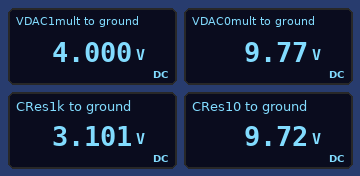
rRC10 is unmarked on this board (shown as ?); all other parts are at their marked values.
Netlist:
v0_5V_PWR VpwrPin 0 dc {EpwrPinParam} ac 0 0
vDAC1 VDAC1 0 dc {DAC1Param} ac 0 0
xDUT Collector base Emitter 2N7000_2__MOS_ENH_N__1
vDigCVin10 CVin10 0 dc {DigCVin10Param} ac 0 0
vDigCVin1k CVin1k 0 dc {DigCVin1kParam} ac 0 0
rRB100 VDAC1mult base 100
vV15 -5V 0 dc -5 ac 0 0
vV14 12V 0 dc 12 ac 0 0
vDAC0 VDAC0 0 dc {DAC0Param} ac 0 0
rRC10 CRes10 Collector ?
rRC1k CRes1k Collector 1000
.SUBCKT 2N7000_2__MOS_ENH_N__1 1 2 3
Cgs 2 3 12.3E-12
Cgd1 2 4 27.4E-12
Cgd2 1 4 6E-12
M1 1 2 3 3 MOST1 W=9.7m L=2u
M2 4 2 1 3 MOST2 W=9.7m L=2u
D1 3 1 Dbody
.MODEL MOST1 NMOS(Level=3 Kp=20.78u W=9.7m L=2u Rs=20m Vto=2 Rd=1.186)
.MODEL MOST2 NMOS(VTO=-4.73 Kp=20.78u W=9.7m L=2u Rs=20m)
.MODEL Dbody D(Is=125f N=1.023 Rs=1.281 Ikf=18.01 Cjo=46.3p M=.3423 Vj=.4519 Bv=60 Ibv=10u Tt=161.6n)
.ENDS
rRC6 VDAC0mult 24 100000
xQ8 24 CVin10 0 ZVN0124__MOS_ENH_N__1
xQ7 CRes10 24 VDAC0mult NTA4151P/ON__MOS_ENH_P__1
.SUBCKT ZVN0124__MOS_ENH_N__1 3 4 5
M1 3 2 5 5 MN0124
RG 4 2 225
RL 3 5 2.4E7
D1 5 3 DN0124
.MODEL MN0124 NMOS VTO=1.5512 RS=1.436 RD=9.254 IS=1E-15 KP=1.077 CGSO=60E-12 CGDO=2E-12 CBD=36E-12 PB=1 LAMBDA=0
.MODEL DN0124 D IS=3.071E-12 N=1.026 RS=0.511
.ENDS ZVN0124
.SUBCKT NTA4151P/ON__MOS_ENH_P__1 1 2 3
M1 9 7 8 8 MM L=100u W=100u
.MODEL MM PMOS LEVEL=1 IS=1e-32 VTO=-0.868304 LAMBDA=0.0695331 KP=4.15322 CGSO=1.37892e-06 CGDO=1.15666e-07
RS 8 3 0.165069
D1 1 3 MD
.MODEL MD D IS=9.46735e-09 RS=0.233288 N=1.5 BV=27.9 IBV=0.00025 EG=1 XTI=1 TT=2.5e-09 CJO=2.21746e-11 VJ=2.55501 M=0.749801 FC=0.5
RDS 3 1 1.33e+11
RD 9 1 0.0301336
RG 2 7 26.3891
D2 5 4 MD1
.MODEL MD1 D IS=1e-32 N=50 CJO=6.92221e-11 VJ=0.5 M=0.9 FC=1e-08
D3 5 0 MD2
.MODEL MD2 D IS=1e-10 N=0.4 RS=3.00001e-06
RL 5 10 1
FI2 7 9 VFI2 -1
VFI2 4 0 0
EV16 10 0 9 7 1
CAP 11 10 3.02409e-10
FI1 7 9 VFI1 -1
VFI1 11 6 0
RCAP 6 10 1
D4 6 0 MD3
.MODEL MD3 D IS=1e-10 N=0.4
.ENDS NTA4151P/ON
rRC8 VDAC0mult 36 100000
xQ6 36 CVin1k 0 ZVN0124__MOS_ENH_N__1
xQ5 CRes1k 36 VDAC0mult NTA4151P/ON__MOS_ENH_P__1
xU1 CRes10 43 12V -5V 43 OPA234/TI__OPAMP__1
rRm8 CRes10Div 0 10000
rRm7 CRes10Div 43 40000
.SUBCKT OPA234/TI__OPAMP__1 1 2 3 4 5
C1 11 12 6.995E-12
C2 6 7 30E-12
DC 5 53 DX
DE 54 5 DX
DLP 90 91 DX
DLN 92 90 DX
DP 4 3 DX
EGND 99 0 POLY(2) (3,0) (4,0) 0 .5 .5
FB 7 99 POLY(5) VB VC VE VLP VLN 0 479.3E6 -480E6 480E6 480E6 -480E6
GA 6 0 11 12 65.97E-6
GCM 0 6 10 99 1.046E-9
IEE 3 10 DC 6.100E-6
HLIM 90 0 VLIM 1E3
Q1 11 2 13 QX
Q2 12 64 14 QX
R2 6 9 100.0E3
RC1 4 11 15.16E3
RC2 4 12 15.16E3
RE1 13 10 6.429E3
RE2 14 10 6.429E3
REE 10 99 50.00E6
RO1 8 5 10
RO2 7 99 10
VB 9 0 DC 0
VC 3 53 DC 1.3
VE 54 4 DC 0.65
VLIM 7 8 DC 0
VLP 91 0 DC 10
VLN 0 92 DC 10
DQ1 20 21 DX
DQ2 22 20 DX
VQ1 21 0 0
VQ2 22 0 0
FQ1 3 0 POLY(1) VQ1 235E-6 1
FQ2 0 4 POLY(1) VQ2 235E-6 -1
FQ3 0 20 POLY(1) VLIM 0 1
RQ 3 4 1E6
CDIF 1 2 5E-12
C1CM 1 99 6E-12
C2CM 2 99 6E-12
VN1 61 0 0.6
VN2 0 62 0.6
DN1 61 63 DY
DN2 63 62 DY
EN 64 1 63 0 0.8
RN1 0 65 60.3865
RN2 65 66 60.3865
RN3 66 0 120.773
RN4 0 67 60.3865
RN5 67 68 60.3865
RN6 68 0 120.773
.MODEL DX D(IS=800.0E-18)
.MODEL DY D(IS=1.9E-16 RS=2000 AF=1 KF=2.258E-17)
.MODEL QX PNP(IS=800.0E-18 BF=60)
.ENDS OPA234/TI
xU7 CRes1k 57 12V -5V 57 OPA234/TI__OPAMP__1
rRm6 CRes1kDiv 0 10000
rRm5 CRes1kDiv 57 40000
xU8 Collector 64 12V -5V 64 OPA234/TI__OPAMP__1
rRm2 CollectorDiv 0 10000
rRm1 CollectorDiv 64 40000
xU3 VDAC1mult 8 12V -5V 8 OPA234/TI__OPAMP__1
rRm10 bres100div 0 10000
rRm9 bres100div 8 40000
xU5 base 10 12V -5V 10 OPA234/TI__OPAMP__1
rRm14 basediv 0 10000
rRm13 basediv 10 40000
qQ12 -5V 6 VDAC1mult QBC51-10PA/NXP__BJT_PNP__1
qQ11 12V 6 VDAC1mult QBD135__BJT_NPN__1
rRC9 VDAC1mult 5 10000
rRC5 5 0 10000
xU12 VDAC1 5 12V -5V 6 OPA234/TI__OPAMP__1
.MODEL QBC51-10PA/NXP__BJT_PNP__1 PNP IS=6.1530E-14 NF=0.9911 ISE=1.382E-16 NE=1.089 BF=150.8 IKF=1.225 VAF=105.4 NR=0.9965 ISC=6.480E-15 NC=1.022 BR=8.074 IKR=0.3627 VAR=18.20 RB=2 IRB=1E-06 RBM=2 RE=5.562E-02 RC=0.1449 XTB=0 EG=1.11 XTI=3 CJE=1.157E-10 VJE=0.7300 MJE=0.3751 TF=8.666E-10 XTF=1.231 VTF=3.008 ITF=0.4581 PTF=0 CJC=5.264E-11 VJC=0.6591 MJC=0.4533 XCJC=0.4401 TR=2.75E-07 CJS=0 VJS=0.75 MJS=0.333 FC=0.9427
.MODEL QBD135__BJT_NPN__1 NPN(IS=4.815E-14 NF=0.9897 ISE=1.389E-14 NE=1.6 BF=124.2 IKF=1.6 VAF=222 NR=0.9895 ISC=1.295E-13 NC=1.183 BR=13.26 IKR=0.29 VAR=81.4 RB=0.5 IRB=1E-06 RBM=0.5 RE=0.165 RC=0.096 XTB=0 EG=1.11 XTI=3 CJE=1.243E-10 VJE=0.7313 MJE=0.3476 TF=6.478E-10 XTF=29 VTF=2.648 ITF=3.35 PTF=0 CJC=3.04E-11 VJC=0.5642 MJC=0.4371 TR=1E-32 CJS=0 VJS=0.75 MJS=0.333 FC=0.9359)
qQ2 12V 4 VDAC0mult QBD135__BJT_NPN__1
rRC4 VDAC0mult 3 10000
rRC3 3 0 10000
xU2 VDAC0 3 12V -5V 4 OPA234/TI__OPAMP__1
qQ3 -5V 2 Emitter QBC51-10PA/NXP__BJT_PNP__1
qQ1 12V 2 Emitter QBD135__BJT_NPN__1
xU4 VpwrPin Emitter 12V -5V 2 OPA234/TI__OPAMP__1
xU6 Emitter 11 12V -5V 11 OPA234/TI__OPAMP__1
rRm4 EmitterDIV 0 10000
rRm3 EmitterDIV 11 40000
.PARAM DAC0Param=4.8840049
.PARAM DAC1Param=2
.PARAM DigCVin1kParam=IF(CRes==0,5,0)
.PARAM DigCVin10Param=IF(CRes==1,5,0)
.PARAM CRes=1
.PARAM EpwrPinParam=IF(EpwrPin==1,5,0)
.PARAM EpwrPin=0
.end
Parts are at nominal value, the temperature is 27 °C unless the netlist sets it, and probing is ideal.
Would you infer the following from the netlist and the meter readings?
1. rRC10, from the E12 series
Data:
33 Ω
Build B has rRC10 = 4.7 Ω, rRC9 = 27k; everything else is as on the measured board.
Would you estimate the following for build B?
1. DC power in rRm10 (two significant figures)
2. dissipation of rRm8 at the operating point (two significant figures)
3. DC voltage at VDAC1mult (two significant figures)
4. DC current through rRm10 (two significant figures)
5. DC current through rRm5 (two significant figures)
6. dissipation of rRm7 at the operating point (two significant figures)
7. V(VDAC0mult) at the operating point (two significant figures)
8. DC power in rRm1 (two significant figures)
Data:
220 µW
200 µW
7.4 V
150 µA
60 µA
810 µW
7.3 V
150 µW
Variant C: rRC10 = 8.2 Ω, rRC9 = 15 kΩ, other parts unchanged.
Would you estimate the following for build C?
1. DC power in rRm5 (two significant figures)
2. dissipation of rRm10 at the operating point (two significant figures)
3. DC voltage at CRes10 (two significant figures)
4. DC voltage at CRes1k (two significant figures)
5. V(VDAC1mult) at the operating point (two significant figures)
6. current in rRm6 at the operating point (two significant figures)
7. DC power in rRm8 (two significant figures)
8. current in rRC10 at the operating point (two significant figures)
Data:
570 µW
100 µW
9.7 V
6.0 V
5.0 V
120 µA
370 µW
450 mA
